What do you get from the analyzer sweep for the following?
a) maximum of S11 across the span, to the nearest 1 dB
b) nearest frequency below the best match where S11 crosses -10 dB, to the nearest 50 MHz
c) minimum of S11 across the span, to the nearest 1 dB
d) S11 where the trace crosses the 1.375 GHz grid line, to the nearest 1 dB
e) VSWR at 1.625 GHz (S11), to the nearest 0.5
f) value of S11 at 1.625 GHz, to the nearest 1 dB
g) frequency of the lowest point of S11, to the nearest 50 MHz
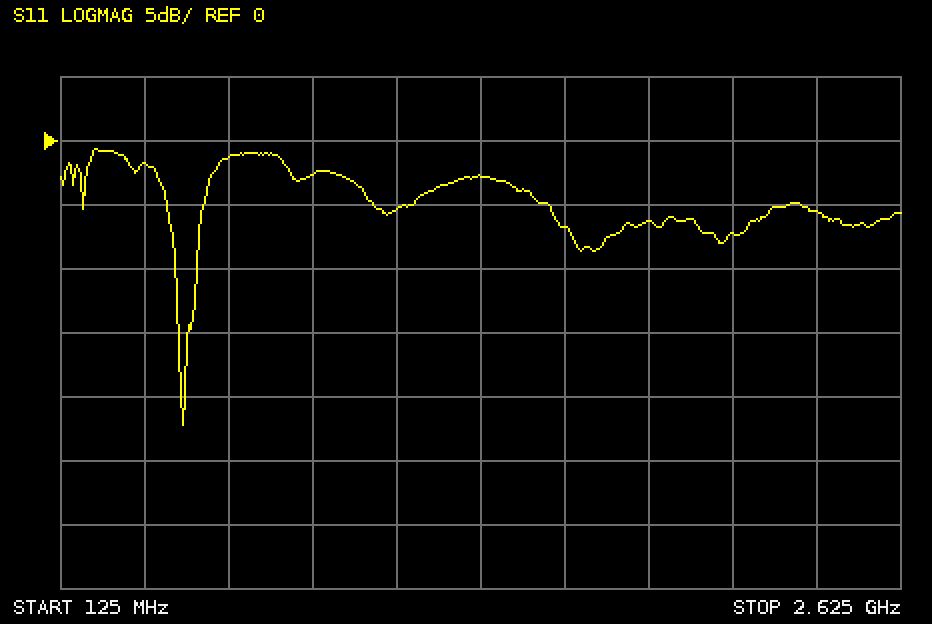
-1 dB
450 MHz
-22 dB
-3 dB
2.5
-7 dB
500 MHz
